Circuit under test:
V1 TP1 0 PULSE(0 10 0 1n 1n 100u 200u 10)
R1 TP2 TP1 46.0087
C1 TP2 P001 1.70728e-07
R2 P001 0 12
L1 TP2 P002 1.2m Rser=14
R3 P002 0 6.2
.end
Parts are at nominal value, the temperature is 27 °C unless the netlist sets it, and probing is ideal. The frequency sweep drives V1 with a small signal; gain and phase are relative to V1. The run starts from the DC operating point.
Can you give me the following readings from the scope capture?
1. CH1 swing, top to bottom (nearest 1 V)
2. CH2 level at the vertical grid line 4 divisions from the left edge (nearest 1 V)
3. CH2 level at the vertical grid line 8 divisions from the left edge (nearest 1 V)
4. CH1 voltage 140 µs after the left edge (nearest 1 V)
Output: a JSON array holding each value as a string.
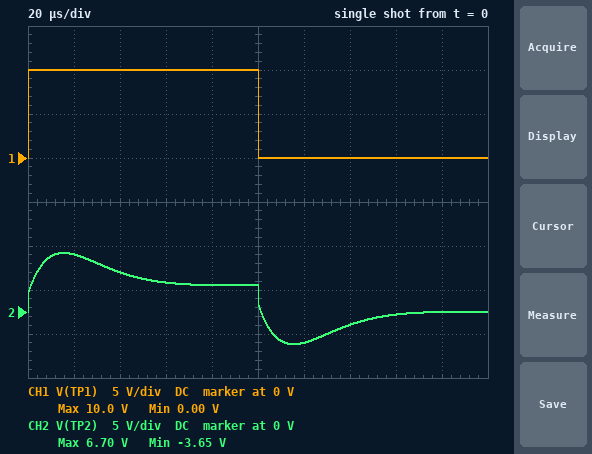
["10 V", "3 V", "0 V", "0 V"]
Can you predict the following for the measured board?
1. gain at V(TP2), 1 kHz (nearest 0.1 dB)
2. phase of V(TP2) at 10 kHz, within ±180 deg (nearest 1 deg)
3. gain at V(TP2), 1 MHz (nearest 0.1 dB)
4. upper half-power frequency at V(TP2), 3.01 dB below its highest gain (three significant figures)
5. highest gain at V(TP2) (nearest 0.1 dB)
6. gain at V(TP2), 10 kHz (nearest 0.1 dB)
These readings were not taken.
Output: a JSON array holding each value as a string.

["-9.8 dB", "4 deg", "-13.7 dB", "26.3 kHz", "-1.6 dB", "-1.7 dB"]
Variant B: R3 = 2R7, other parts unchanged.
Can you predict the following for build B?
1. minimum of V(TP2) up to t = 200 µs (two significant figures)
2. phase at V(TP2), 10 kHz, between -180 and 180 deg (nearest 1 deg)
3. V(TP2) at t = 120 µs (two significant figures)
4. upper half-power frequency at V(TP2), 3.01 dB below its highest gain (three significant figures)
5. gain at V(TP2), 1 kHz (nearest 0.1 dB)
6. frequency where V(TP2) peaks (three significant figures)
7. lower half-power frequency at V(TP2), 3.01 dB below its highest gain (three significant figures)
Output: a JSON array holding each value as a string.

["-4.0 V", "5 deg", "-3.8 V", "25.8 kHz", "-10.7 dB", "11.4 kHz", "4.95 kHz"]
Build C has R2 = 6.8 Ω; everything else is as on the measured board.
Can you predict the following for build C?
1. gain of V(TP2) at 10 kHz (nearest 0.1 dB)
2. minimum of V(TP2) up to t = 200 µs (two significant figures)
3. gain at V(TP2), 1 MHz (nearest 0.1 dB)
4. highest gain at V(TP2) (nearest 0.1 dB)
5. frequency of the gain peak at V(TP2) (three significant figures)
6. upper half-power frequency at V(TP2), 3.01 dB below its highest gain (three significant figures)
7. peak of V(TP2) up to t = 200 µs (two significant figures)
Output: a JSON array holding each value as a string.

["-1.5 dB", "-3.9 V", "-17.7 dB", "-1.3 dB", "12.1 kHz", "26.8 kHz", "6.9 V"]
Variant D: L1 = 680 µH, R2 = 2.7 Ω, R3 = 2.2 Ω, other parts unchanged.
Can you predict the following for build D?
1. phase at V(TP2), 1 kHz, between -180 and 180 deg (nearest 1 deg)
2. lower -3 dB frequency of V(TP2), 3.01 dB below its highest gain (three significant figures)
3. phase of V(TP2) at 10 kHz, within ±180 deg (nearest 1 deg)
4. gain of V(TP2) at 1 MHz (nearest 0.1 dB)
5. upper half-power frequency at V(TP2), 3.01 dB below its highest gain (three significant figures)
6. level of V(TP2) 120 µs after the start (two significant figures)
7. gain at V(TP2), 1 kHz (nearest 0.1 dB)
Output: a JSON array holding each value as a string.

["10 deg", "7.95 kHz", "18 deg", "-24.6 dB", "31.6 kHz", "-3.0 V", "-11.4 dB"]
